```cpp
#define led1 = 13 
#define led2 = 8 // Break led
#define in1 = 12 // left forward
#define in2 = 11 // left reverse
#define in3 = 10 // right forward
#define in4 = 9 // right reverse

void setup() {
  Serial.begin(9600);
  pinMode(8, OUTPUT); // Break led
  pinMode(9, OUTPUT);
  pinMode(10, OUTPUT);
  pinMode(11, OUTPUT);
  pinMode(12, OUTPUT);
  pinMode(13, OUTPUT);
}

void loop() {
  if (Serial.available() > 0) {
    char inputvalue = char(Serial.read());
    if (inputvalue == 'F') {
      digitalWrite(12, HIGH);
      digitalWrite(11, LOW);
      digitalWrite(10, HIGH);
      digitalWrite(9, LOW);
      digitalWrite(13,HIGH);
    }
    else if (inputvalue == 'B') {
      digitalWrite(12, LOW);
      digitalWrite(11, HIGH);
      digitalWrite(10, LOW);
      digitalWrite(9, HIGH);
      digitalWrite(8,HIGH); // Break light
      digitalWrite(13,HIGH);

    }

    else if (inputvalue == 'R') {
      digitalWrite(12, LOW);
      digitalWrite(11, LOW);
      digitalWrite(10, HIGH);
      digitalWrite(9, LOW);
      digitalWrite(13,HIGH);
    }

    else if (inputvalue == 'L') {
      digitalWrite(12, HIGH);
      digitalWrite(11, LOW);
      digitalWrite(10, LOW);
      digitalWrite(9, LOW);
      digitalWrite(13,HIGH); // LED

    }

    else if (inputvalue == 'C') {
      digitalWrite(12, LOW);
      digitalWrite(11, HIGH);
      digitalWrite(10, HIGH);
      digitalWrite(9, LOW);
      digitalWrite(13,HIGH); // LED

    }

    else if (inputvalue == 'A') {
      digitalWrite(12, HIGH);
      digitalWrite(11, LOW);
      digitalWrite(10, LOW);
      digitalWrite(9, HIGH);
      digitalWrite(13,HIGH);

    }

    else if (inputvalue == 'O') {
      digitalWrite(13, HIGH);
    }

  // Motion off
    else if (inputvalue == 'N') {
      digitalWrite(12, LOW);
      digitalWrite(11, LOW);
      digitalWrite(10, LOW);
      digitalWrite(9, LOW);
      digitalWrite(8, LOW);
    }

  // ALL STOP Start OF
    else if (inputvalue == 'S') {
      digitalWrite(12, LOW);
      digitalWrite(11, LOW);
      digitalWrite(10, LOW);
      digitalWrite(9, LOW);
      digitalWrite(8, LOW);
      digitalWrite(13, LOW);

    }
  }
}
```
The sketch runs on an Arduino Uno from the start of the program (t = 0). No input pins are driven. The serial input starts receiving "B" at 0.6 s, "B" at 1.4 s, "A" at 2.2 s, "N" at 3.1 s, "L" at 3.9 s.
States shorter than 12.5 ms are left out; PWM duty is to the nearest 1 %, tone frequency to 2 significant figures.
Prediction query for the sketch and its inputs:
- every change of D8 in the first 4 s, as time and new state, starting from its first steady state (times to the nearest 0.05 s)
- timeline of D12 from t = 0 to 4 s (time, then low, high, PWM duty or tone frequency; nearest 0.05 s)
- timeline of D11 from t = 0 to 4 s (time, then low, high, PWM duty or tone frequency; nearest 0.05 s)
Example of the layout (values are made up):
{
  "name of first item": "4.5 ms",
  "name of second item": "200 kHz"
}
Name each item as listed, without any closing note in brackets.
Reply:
{
  "every change of D8 in the first 4 s, as time and new state, starting from its first steady state": "0 s low; 0.6 s high; 3.1 s low",
  "timeline of D12 from t = 0 to 4 s": "0 s low; 2.2 s high; 3.1 s low; 3.9 s high",
  "timeline of D11 from t = 0 to 4 s": "0 s low; 0.6 s high; 2.2 s low"
}
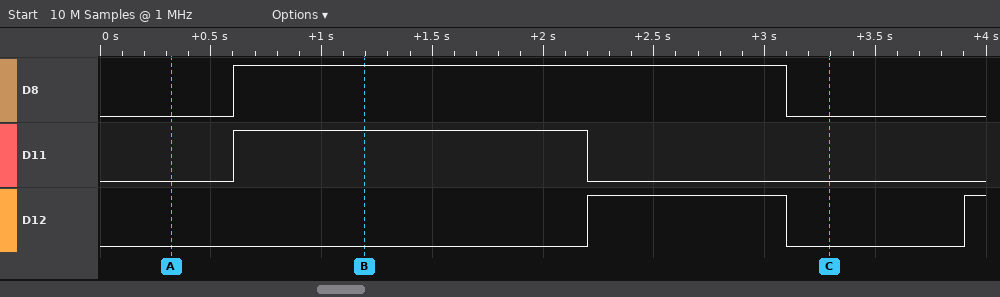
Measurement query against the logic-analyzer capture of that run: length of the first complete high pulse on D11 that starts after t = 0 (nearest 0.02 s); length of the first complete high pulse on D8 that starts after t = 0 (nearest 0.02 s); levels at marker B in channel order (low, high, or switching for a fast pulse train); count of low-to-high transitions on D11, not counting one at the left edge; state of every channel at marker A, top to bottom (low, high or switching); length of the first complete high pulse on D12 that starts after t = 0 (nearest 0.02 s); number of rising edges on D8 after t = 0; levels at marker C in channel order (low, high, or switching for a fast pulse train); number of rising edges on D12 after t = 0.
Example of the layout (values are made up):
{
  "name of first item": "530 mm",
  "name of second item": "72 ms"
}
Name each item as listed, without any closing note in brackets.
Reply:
{
  "length of the first complete high pulse on D11 that starts after t = 0": "1.60 s",
  "length of the first complete high pulse on D8 that starts after t = 0": "2.50 s",
  "levels at marker B in channel order": "D8 high, D11 high, D12 low",
  "count of low-to-high transitions on D11, not counting one at the left edge": "1",
  "state of every channel at marker A, top to bottom": "D8 low, D11 low, D12 low",
  "length of the first complete high pulse on D12 that starts after t = 0": "0.90 s",
  "number of rising edges on D8 after t = 0": "1",
  "levels at marker C in channel order": "D8 low, D11 low, D12 low",
  "number of rising edges on D12 after t = 0": "2"
}
